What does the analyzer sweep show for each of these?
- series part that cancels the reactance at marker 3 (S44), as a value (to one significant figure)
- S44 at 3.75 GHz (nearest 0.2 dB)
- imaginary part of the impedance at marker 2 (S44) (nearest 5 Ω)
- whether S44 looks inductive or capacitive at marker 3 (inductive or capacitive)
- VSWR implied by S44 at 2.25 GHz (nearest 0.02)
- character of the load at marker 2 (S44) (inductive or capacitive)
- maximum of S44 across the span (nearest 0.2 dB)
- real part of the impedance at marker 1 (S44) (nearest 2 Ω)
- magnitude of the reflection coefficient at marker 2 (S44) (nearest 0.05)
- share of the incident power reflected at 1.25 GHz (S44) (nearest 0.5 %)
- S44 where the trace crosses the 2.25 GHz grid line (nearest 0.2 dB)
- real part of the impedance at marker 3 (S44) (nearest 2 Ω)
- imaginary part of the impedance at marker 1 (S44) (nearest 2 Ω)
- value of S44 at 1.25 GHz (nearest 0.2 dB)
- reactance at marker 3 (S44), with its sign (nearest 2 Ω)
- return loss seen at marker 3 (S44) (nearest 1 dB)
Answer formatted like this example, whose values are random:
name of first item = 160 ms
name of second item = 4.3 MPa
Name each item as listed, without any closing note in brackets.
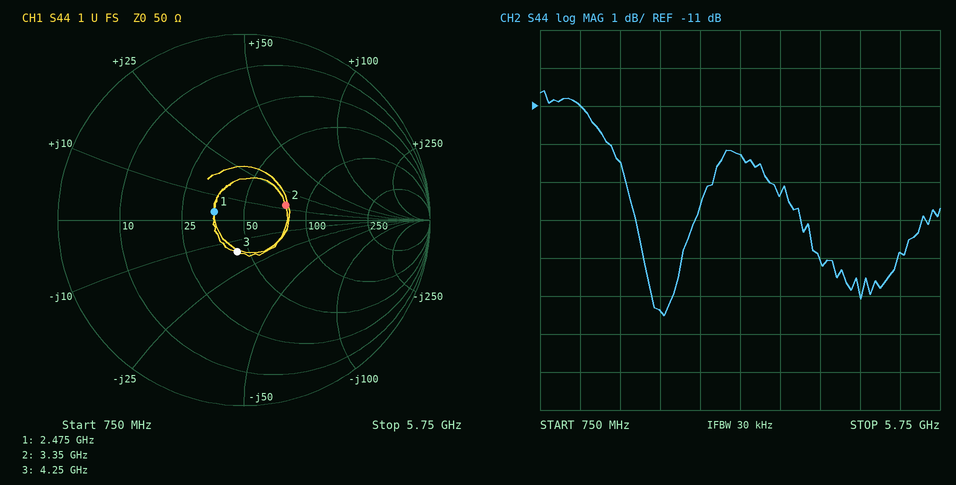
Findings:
series part that cancels the reactance at marker 3 (S44), as a value = 600 pH
S44 at 3.75 GHz = -13.4 dB
imaginary part of the impedance at marker 2 (S44) = +15 Ω
whether S44 looks inductive or capacitive at marker 3 = capacitive
VSWR implied by S44 at 2.25 GHz = 1.36
character of the load at marker 2 (S44) = inductive
maximum of S44 across the span = -10.6 dB
real part of the impedance at marker 1 (S44) = 36 Ω
magnitude of the reflection coefficient at marker 2 (S44) = 0.25
share of the incident power reflected at 1.25 GHz (S44) = 8.0 %
S44 where the trace crosses the 2.25 GHz grid line = -16.4 dB
real part of the impedance at marker 3 (S44) = 44 Ω
imaginary part of the impedance at marker 1 (S44) = +4 Ω
value of S44 at 1.25 GHz = -11.0 dB
reactance at marker 3 (S44), with its sign = -16 Ω
return loss seen at marker 3 (S44) = 15 dB
